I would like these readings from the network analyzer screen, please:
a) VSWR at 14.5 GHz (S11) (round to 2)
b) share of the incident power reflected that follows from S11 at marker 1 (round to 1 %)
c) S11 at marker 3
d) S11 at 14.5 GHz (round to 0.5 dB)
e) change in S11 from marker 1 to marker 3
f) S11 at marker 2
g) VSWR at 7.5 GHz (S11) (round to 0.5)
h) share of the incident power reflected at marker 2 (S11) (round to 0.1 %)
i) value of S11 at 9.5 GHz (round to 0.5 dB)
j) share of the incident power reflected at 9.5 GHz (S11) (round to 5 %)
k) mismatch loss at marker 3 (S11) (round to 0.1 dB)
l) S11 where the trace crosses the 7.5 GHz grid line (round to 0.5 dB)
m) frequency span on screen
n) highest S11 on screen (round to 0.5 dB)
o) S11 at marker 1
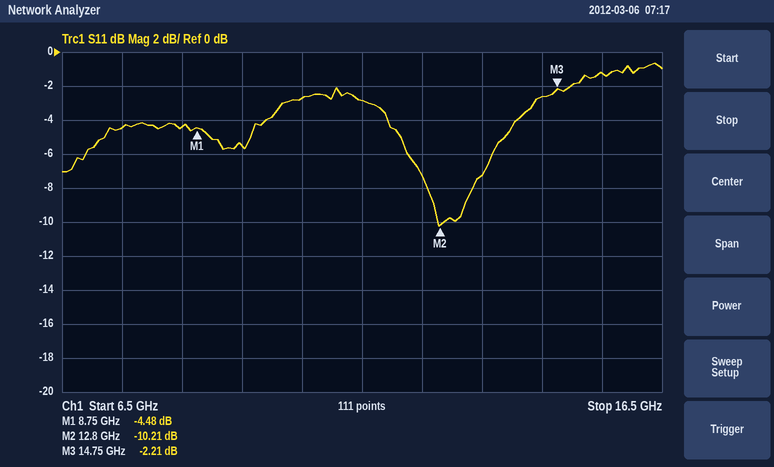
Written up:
6
36 %
-2.21 dB
-2.5 dB
2.27 dB
-10.21 dB
4.0
9.5 %
-5.5 dB
30 %
4.0 dB
-4.5 dB
10 GHz
-0.5 dB
-4.48 dB
